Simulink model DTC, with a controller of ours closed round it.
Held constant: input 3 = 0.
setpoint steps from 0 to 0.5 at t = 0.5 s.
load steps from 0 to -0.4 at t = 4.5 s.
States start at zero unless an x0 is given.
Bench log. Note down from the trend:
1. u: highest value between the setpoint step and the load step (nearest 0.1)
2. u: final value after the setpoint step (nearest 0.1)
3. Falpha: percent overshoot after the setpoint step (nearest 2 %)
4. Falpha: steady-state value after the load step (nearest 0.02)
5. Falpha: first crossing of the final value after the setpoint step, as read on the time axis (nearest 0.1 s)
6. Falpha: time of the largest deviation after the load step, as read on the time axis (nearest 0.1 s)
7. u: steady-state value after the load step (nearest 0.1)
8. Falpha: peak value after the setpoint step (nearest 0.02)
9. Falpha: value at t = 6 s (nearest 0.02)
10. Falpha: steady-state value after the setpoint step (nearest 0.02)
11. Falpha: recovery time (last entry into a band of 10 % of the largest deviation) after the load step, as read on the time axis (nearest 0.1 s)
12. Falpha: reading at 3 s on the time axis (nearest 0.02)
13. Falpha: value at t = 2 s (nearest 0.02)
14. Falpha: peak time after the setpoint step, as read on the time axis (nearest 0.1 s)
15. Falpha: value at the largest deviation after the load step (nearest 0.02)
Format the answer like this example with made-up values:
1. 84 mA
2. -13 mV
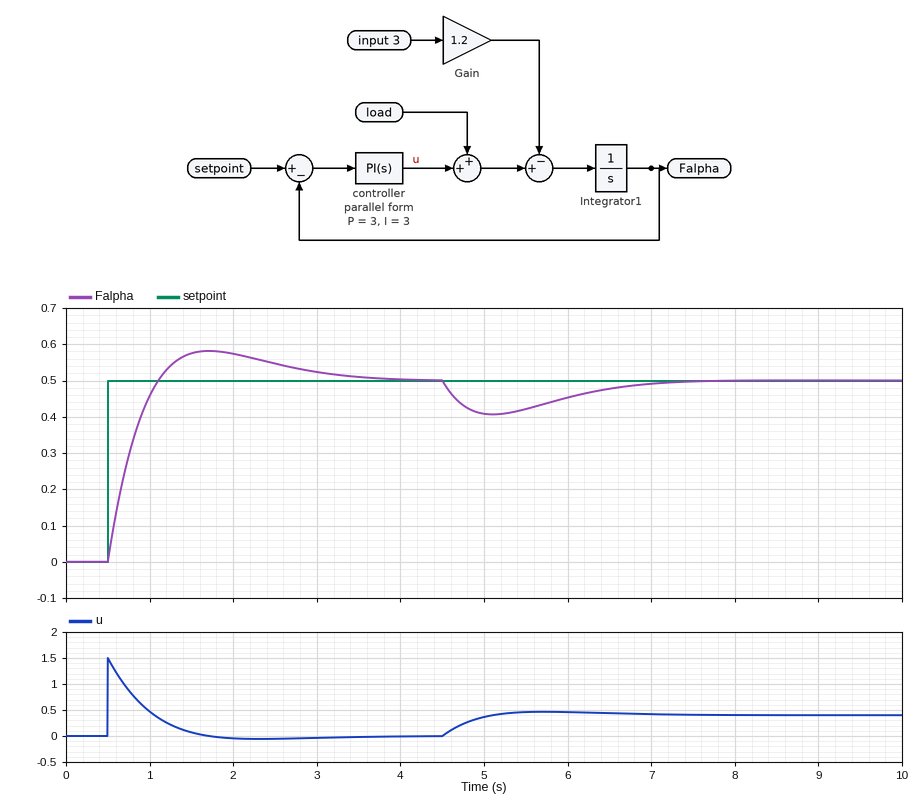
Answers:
1. 1.5
2. 0.0
3. 16 %
4. 0.50
5. 1.1 s
6. 5.1 s
7. 0.4
8. 0.58
9. 0.46
10. 0.50
11. 7.0 s
12. 0.52
13. 0.58
14. 1.7 s
15. 0.40
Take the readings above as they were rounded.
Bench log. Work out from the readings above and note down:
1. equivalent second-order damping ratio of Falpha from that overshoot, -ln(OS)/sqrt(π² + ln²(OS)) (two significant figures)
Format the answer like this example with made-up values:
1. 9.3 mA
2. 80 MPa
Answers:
1. 0.50
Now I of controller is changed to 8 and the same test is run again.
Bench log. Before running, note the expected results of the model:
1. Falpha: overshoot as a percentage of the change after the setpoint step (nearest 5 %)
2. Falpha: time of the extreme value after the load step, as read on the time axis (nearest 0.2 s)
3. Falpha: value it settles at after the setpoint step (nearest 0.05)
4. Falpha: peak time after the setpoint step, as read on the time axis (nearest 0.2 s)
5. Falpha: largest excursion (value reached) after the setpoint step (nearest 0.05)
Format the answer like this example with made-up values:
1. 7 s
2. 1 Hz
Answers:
1. 30 %
2. 5.0 s
3. 0.50
4. 1.4 s
5. 0.65
